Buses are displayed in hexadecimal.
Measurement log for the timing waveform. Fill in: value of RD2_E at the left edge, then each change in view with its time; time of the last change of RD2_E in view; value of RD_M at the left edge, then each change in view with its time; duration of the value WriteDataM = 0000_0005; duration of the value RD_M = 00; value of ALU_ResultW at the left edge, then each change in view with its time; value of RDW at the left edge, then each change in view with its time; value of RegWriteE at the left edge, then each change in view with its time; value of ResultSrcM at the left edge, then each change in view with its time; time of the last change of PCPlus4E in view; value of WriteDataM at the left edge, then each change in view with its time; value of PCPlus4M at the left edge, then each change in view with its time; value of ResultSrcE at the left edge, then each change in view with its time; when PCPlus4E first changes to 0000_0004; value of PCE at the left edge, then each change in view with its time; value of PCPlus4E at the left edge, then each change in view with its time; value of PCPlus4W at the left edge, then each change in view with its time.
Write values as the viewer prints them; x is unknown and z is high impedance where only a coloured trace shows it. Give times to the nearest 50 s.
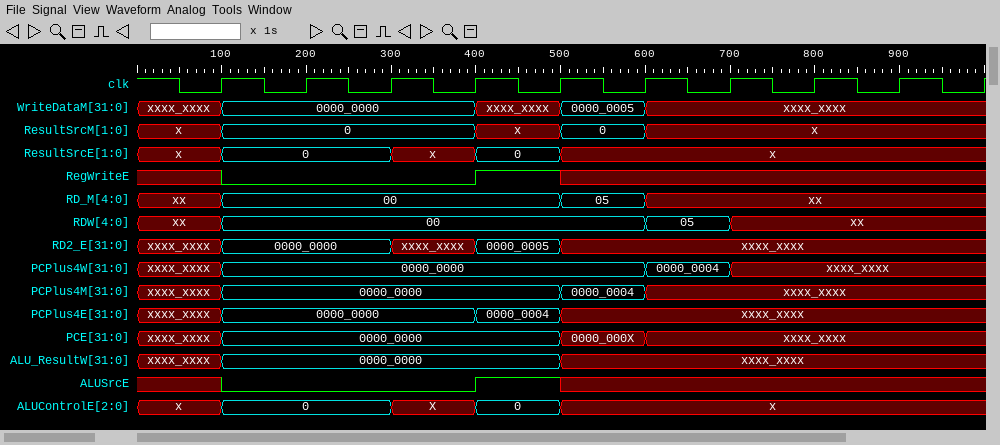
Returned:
xxxx_xxxx, 0000_0000 at 100 s, xxxx_xxxx at 300 s, 0000_0005 at 400 s, xxxx_xxxx at 500 s
500 s
xx, 00 at 100 s, 05 at 500 s, xx at 600 s
100 s
400 s
xxxx_xxxx, 0000_0000 at 100 s, xxxx_xxxx at 500 s
xx, 00 at 100 s, 05 at 600 s, xx at 700 s
x, 0 at 100 s, 1 at 400 s, x at 500 s
x, 0 at 100 s, x at 400 s, 0 at 500 s, x at 600 s
500 s
xxxx_xxxx, 0000_0000 at 100 s, xxxx_xxxx at 400 s, 0000_0005 at 500 s, xxxx_xxxx at 600 s
xxxx_xxxx, 0000_0000 at 100 s, 0000_0004 at 500 s, xxxx_xxxx at 600 s
x, 0 at 100 s, x at 300 s, 0 at 400 s, x at 500 s
400 s
xxxx_xxxx, 0000_0000 at 100 s, 0000_000X at 500 s, xxxx_xxxx at 600 s
xxxx_xxxx, 0000_0000 at 100 s, 0000_0004 at 400 s, xxxx_xxxx at 500 s
xxxx_xxxx, 0000_0000 at 100 s, 0000_0004 at 600 s, xxxx_xxxx at 700 s
